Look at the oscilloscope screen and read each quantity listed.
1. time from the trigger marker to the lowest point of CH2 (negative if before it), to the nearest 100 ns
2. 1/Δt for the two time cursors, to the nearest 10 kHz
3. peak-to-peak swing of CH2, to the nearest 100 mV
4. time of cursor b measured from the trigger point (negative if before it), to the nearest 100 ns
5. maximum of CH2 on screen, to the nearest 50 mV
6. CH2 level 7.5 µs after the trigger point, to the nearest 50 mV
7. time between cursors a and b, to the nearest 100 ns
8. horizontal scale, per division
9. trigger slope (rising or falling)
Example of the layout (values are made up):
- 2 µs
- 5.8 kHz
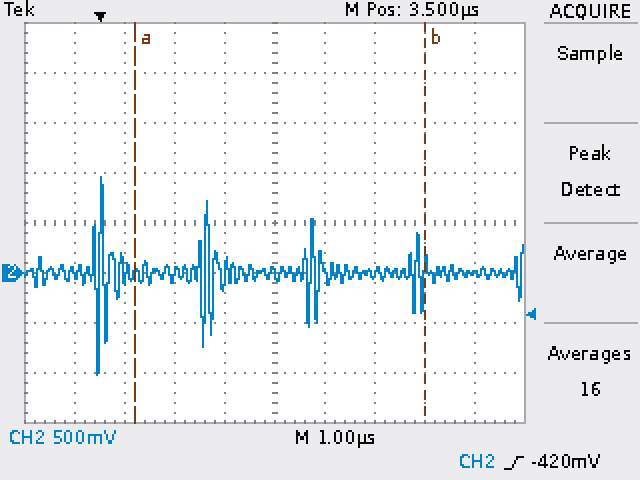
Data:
- 0.0 µs
- 170 kHz
- 2.00 V
- +6.5 µs
- 950 mV
- 0 mV
- 5.8 µs
- 1 µs
- rising
